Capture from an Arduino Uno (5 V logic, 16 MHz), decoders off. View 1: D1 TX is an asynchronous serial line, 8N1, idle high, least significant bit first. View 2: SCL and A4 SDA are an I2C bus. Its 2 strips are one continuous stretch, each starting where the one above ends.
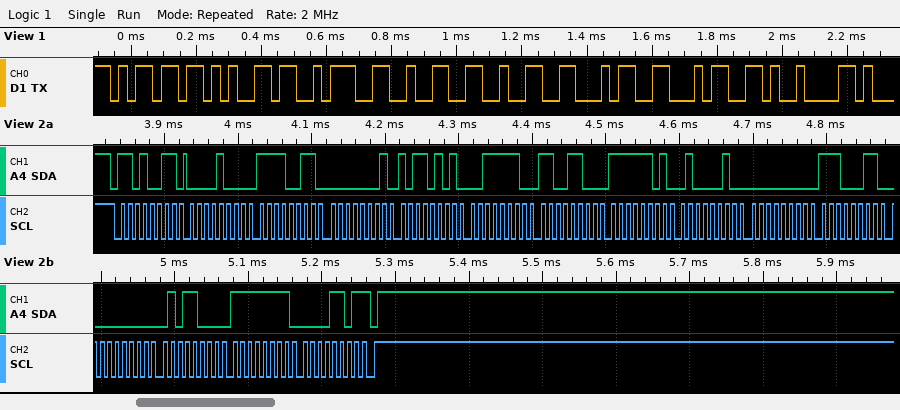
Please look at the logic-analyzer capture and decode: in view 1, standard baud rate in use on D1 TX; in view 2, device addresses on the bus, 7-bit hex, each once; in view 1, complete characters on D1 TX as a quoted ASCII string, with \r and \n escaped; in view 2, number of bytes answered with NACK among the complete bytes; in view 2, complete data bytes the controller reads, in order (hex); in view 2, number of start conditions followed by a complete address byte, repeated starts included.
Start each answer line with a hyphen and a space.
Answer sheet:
- 38400 baud
- 0x69
- "me:2244\t"
- 1
- 08 F3 01 B5 3E CC FD 42 00 E3 00 58 FF 0D
- 1
